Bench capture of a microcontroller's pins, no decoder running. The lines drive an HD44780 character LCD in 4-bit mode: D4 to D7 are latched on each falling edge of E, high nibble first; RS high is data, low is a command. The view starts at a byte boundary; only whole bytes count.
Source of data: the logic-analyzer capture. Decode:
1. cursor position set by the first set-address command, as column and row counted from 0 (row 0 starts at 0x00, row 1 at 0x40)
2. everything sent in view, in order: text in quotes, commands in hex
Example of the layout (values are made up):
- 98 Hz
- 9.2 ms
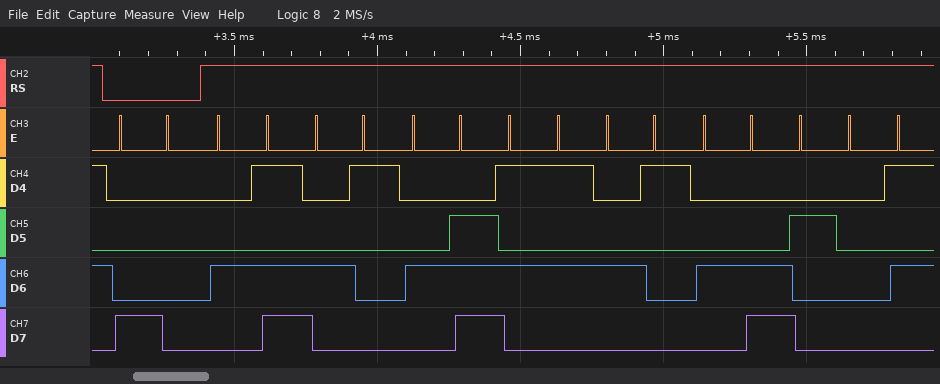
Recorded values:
- column 0, row 0
- 0x80 "MANUAL "
